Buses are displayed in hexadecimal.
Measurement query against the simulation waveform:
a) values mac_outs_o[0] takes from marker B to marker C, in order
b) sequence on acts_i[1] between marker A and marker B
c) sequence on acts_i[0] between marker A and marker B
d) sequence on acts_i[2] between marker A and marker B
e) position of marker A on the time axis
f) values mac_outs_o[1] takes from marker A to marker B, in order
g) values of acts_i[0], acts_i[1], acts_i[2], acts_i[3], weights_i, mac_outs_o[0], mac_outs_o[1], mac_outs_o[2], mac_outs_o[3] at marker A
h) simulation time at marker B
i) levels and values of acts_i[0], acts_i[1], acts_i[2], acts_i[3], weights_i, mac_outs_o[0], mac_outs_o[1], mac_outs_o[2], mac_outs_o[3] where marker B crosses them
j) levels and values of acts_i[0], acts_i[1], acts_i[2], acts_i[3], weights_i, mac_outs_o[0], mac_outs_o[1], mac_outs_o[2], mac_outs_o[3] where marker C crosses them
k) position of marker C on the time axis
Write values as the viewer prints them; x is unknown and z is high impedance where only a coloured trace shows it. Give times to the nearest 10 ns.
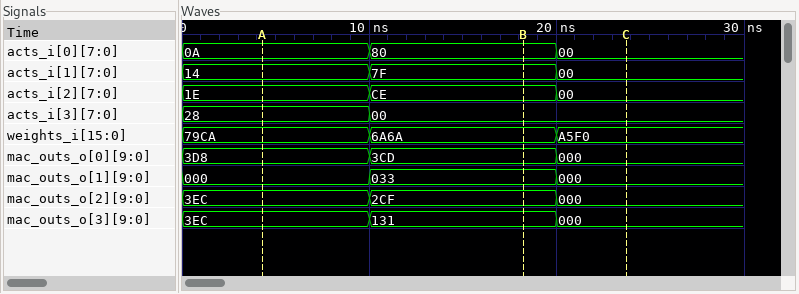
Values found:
3CD, 000
14, 7F
0A, 80
1E, CE
0 ns
000, 033
acts_i[0]=0A, acts_i[1]=14, acts_i[2]=1E, acts_i[3]=28, weights_i=79CA, mac_outs_o[0]=3D8, mac_outs_o[1]=000, mac_outs_o[2]=3EC, mac_outs_o[3]=3EC
20 ns
acts_i[0]=80, acts_i[1]=7F, acts_i[2]=CE, acts_i[3]=00, weights_i=6A6A, mac_outs_o[0]=3CD, mac_outs_o[1]=033, mac_outs_o[2]=2CF, mac_outs_o[3]=131
acts_i[0]=00, acts_i[1]=00, acts_i[2]=00, acts_i[3]=00, weights_i=A5F0, mac_outs_o[0]=000, mac_outs_o[1]=000, mac_outs_o[2]=000, mac_outs_o[3]=000
20 ns
